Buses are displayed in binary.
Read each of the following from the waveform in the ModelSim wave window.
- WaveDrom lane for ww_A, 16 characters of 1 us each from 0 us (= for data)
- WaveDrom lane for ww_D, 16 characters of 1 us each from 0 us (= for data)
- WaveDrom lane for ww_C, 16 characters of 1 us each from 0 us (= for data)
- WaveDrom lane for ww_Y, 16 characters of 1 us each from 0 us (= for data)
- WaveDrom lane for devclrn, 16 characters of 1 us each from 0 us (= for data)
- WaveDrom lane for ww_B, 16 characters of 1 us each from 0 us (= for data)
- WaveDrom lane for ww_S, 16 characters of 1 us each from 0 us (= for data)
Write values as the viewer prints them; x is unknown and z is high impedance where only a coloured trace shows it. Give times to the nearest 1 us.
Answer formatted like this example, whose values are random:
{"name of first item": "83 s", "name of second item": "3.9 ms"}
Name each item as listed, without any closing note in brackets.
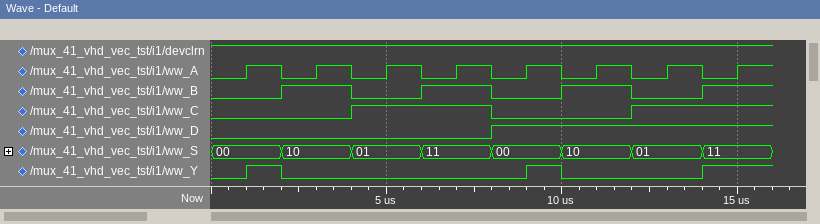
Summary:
{"WaveDrom lane for ww_A, 16 characters of 1 us each from 0 us": "{name: 'ww_A', wave: '0101010101010101'}", "WaveDrom lane for ww_D, 16 characters of 1 us each from 0 us": "{name: 'ww_D', wave: '0.......1.......'}", "WaveDrom lane for ww_C, 16 characters of 1 us each from 0 us": "{name: 'ww_C', wave: '0...1...0...1...'}", "WaveDrom lane for ww_Y, 16 characters of 1 us each from 0 us": "{name: 'ww_Y', wave: '010......10...1.'}", "WaveDrom lane for devclrn, 16 characters of 1 us each from 0 us": "{name: 'devclrn', wave: '1...............'}", "WaveDrom lane for ww_B, 16 characters of 1 us each from 0 us": "{name: 'ww_B', wave: '0.1.0.1.0.1.0.1.'}", "WaveDrom lane for ww_S, 16 characters of 1 us each from 0 us": "{name: 'ww_S', wave: '=.=.=.=.=.=.=.=.', data: '00 10 01 11 00 10 01 11'}"}
